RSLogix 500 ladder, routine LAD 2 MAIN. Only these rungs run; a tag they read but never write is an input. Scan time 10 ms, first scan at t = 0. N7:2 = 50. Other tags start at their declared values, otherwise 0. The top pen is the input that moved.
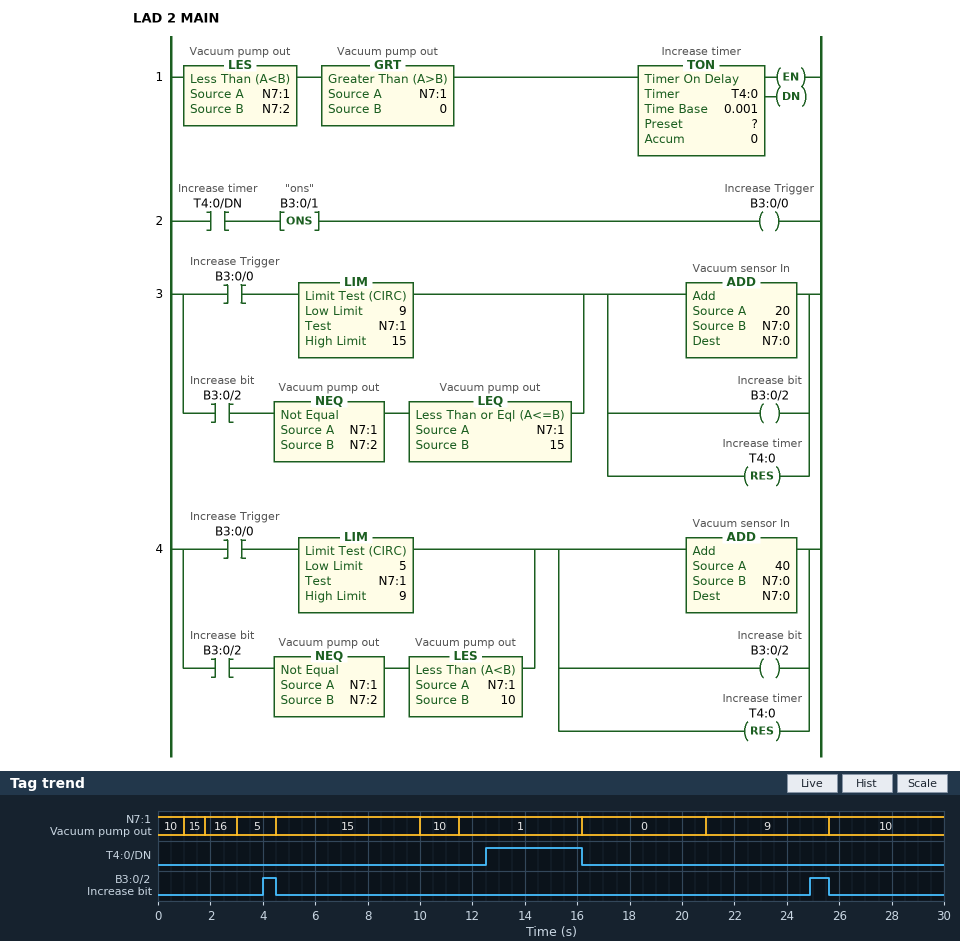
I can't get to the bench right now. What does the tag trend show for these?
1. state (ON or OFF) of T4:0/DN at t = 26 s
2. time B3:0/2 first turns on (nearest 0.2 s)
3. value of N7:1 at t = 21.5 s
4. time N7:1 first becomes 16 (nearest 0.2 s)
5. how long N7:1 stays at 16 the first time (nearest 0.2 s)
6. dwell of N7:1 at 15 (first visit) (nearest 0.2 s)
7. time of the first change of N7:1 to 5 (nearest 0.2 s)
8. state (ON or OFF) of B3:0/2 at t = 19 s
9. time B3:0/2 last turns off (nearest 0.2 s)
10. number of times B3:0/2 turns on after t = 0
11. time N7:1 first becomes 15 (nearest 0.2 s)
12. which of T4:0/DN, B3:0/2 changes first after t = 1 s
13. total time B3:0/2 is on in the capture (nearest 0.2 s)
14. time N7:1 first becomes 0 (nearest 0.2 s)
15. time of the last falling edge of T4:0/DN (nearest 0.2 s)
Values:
OFF
4.0 s
9
1.8 s
1.2 s
0.8 s
3.0 s
OFF
25.6 s
2
1.0 s
B3:0/2
1.2 s
16.2 s
16.2 s
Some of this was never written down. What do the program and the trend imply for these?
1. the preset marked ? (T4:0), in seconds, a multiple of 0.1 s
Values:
4.0 s
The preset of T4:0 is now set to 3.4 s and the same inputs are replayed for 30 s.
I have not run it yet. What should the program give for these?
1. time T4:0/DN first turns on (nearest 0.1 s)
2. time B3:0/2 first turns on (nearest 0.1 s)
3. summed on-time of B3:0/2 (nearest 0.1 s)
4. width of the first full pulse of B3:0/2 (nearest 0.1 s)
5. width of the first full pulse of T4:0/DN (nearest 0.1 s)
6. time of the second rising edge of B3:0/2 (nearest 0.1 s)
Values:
14.7 s
3.4 s
2.4 s
1.1 s
1.5 s
24.3 s
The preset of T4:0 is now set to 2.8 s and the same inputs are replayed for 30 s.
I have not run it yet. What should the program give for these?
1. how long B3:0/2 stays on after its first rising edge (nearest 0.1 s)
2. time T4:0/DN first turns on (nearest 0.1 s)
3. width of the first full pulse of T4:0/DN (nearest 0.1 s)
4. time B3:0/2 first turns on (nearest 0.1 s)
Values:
1.9 s
2.8 s
13.4 s
23.7 s
